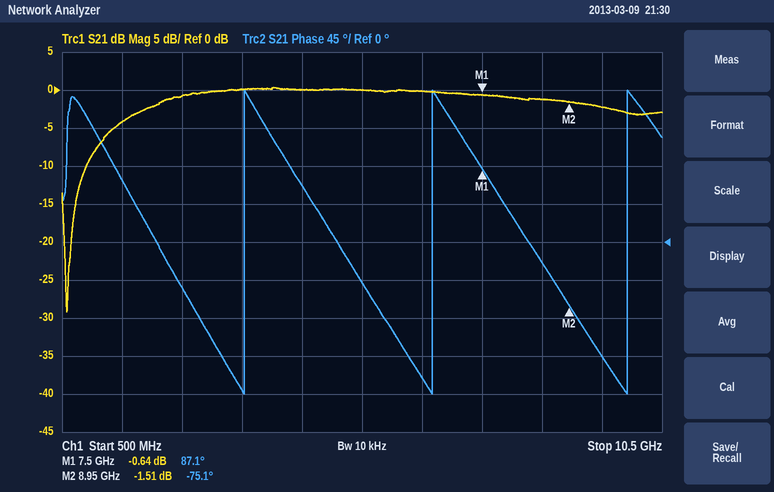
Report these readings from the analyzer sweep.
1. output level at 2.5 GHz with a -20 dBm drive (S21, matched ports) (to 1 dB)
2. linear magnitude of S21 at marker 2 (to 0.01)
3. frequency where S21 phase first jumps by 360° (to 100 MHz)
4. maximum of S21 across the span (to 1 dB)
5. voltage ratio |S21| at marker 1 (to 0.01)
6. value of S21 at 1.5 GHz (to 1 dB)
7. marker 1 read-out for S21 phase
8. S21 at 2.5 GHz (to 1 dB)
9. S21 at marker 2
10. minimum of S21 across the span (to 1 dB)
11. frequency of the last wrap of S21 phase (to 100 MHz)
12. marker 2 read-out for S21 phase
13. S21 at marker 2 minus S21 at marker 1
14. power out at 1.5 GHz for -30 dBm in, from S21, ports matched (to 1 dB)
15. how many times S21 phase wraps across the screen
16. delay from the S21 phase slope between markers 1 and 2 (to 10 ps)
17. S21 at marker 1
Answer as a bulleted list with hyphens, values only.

- -21 dBm
- 0.84
- 3.5 GHz
- 0 dB
- 0.93
- -4 dB
- 87.1°
- -1 dB
- -1.51 dB
- -29 dB
- 9.9 GHz
- -75.1°
- -0.87 dB
- -34 dBm
- 3
- 310 ps
- -0.64 dB
